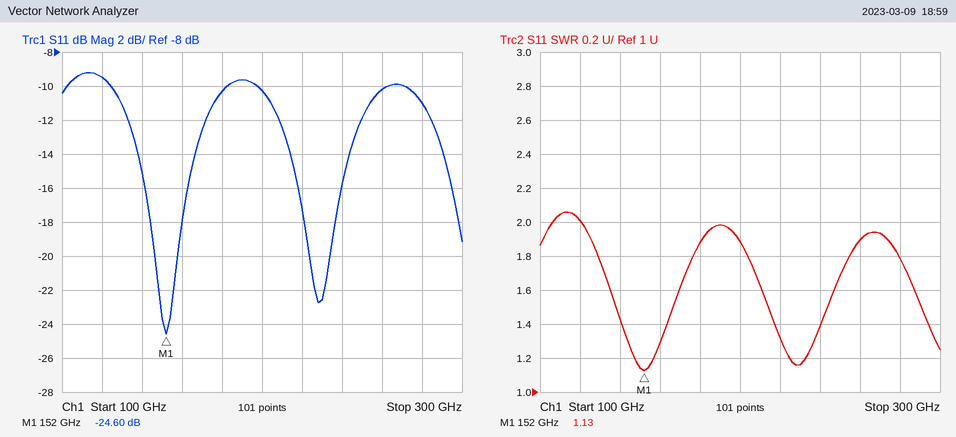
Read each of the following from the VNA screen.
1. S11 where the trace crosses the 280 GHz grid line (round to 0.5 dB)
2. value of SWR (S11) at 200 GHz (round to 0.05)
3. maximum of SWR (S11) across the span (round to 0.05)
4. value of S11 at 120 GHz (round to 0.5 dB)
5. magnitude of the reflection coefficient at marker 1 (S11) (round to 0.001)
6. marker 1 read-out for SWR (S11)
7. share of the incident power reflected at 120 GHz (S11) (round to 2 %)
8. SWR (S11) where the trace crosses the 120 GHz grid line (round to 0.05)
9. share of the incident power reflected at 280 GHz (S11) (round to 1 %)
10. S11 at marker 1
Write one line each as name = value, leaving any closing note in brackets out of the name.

S11 where the trace crosses the 280 GHz grid line = -11.0 dB
value of SWR (S11) at 200 GHz = 1.90
maximum of SWR (S11) across the span = 2.05
value of S11 at 120 GHz = -9.5 dB
magnitude of the reflection coefficient at marker 1 (S11) = 0.059
marker 1 read-out for SWR = 1.13
share of the incident power reflected at 120 GHz (S11) = 12 %
SWR (S11) where the trace crosses the 120 GHz grid line = 2.00
share of the incident power reflected at 280 GHz (S11) = 8 %
S11 at marker 1 = -24.60 dB
